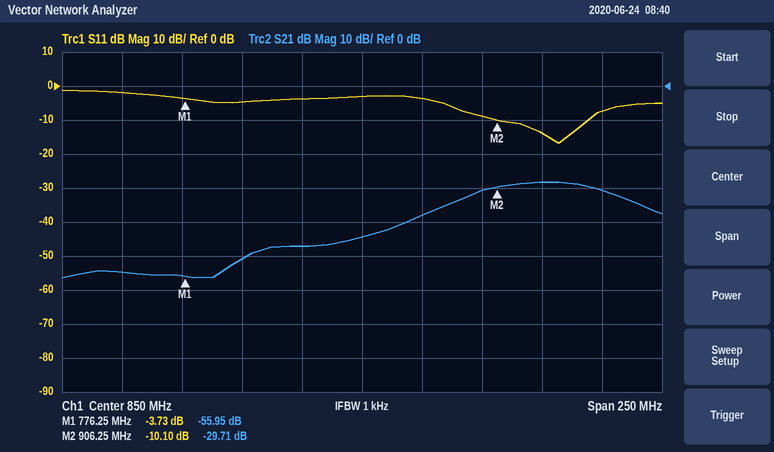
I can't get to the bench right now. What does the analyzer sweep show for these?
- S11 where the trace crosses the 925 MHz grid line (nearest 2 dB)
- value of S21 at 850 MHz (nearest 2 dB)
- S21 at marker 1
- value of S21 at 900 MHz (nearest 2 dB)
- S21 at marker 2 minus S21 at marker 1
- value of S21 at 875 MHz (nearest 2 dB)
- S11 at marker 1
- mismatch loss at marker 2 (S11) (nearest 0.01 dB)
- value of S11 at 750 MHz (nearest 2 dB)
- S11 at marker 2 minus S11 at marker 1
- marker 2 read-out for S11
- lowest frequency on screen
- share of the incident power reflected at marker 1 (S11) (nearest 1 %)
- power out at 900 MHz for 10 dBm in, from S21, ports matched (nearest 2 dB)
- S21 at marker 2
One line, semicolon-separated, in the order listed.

-14 dB; -44 dB; -55.95 dB; -30 dB; 26.24 dB; -38 dB; -3.73 dB; 0.45 dB; -2 dB; -6.37 dB; -10.10 dB; 725 MHz; 42 %; -20 dBm; -29.71 dB
